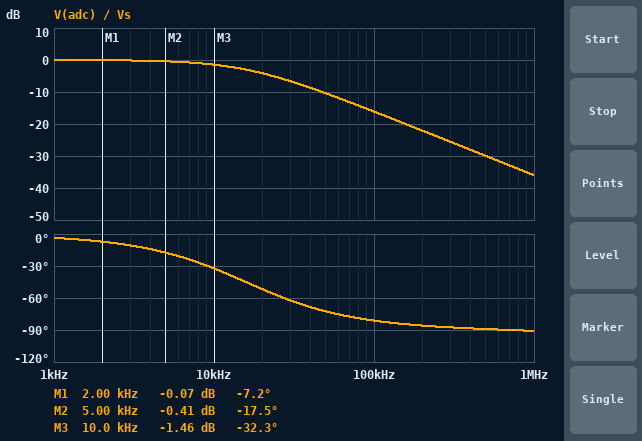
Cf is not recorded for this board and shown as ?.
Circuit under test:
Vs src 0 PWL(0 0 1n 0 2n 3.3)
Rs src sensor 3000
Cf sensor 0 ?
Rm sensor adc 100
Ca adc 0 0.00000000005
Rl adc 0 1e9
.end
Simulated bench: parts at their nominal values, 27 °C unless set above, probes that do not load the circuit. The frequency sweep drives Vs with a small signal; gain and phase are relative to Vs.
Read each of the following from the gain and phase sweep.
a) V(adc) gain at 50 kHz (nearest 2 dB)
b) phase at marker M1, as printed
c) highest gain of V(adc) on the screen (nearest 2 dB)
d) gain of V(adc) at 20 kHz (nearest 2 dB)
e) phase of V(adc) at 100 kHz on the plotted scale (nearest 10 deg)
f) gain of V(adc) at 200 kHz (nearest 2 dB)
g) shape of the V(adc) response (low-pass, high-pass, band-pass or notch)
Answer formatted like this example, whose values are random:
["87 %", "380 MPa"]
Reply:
["-10 dB", "-7.2 deg", "0 dB", "-4 dB", "-80 deg", "-22 dB", "low-pass"]
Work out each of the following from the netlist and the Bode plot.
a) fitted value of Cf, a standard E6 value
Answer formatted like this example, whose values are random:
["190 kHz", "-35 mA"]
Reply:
["3.3 nF"]
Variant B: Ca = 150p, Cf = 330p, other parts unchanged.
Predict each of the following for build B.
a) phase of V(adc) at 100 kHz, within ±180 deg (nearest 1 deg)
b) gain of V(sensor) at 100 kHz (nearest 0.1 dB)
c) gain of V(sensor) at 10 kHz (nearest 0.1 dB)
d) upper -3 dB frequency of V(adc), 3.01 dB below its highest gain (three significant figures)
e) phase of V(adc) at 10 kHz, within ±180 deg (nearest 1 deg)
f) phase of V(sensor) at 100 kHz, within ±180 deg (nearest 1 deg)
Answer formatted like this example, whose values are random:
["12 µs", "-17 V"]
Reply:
["-43 deg", "-2.6 dB", "0 dB", "110 kHz", "-5 deg", "-42 deg"]
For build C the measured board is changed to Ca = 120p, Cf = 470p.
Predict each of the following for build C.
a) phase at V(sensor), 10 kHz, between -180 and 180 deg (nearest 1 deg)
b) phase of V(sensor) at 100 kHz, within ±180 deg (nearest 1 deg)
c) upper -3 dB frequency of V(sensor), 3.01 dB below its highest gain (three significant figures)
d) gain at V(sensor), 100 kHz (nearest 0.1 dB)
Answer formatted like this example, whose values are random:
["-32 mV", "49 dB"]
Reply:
["-6 deg", "-48 deg", "89.8 kHz", "-3.5 dB"]
